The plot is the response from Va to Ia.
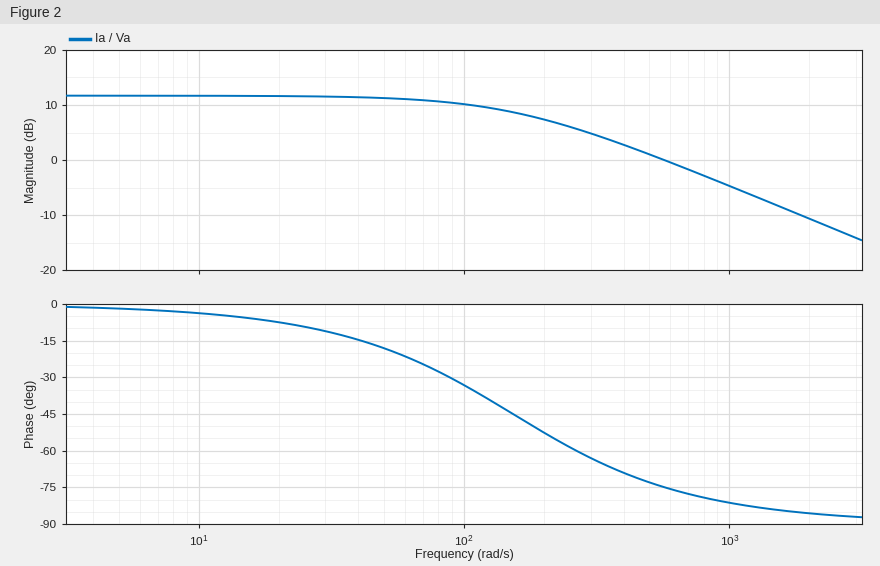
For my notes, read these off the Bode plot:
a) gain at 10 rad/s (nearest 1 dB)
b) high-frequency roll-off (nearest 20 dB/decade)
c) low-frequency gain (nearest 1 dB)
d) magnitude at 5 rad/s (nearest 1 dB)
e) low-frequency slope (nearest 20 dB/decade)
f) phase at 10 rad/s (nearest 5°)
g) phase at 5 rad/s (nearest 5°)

12 dB
-20 dB/decade
12 dB
12 dB
0 dB/decade
-5°
0°
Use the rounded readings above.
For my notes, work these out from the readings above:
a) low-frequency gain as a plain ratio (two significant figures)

4.0
